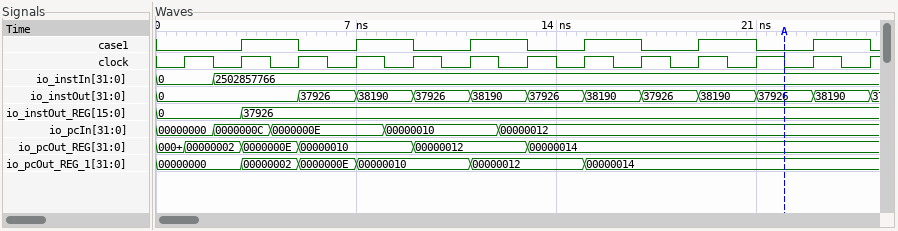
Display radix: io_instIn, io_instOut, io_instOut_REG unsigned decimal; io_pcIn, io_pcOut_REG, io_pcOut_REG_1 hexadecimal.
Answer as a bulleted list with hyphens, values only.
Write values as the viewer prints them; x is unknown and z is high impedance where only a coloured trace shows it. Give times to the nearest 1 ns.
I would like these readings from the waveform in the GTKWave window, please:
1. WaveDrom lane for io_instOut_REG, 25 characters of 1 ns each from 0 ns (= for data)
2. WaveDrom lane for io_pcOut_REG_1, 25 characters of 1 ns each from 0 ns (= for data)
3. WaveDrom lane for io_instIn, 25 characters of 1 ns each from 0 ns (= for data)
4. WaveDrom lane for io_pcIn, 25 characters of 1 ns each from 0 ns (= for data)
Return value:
- {name: 'io_instOut_REG', wave: '=..=.....................', data: '0 37926'}
- {name: 'io_pcOut_REG_1', wave: '=..=.=.=...=...=.........', data: '00000000 00000002 0000000E 00000010 00000012 00000014'}
- {name: 'io_instIn', wave: '=.=......................', data: '0 2502857766'}
- {name: 'io_pcIn', wave: '=.=.=...=...=............', data: '00000000 0000000C 0000000E 00000010 00000012'}
